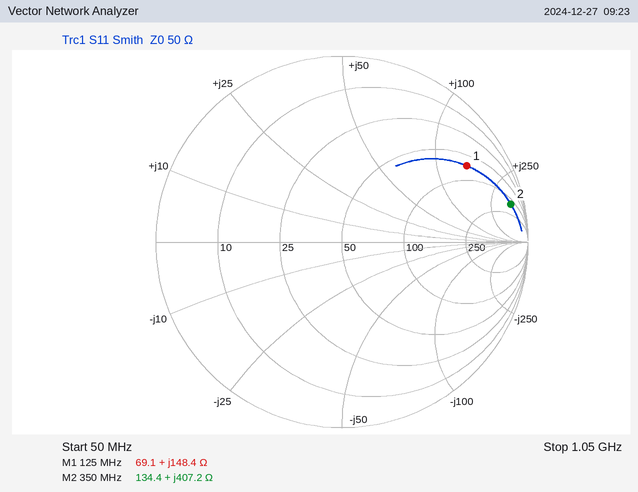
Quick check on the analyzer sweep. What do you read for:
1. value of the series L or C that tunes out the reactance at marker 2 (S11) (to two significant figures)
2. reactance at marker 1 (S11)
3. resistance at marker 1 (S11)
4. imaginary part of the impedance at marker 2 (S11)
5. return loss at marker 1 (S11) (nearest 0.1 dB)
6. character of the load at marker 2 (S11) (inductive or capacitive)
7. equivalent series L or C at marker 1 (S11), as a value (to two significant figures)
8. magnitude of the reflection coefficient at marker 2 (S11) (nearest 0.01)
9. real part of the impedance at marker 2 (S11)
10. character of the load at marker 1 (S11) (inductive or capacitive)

1.1 pF
+148.4 Ω
69.1 Ω
+407.2 Ω
2.1 dB
inductive
190 nH
0.93
134.4 Ω
inductive
